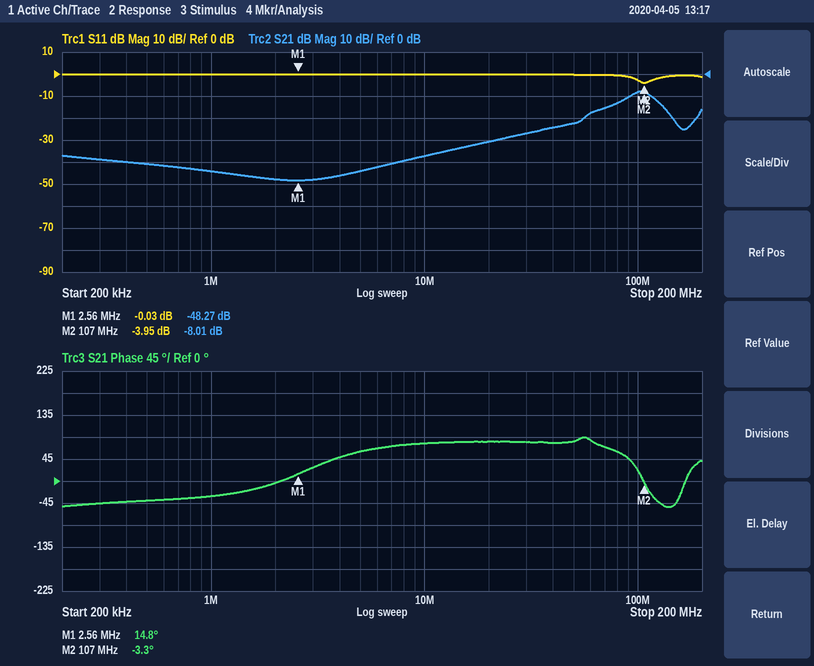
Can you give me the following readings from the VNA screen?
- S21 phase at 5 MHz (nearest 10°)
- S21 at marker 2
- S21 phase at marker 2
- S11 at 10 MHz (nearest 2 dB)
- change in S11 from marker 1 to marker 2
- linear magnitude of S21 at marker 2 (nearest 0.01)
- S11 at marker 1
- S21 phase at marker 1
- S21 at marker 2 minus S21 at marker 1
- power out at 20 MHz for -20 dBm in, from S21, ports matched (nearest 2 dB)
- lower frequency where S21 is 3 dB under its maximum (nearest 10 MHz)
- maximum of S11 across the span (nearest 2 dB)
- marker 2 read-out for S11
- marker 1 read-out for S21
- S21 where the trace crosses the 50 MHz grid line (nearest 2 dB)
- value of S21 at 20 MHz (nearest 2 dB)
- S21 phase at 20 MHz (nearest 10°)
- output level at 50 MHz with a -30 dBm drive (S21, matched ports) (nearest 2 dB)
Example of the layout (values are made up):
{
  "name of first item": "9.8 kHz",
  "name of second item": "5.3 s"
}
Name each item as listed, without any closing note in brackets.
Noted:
{
  "S21 phase at 5 MHz": "60°",
  "S21 at marker 2": "-8.01 dB",
  "S21 phase at marker 2": "-3.3°",
  "S11 at 10 MHz": "0 dB",
  "change in S11 from marker 1 to marker 2": "-3.92 dB",
  "linear magnitude of S21 at marker 2": "0.40",
  "S11 at marker 1": "-0.03 dB",
  "S21 phase at marker 1": "14.8°",
  "S21 at marker 2 minus S21 at marker 1": "40.26 dB",
  "power out at 20 MHz for -20 dBm in, from S21, ports matched": "-50 dBm",
  "lower frequency where S21 is 3 dB under its maximum": "90 MHz",
  "maximum of S11 across the span": "0 dB",
  "marker 2 read-out for S11": "-3.95 dB",
  "marker 1 read-out for S21": "-48.27 dB",
  "S21 where the trace crosses the 50 MHz grid line": "-22 dB",
  "value of S21 at 20 MHz": "-30 dB",
  "S21 phase at 20 MHz": "80°",
  "output level at 50 MHz with a -30 dBm drive (S21, matched ports)": "-52 dBm"
}
